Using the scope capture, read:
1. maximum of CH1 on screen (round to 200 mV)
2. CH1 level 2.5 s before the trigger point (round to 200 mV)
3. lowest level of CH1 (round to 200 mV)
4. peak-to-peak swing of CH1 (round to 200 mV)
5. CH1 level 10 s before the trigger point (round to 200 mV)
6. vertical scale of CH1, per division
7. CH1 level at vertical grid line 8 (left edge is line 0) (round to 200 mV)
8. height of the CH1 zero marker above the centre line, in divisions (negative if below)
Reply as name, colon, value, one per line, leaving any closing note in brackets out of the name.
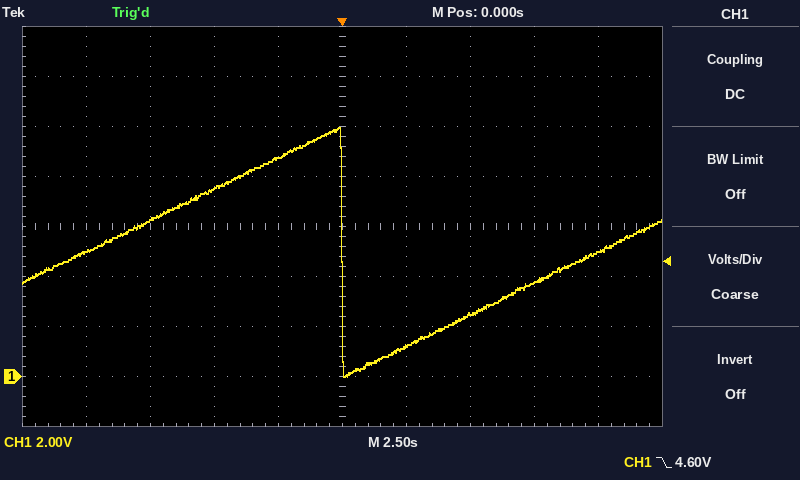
maximum of CH1 on screen: 10.0 V
CH1 level 2.5 s before the trigger point: 8.8 V
lowest level of CH1: 0.0 V
peak-to-peak swing of CH1: 10.0 V
CH1 level 10 s before the trigger point: 5.0 V
vertical scale of CH1, per division: 2 V
CH1 level at vertical grid line 8 (left edge is line 0): 3.8 V
height of the CH1 zero marker above the centre line, in divisions: -3.0 div
